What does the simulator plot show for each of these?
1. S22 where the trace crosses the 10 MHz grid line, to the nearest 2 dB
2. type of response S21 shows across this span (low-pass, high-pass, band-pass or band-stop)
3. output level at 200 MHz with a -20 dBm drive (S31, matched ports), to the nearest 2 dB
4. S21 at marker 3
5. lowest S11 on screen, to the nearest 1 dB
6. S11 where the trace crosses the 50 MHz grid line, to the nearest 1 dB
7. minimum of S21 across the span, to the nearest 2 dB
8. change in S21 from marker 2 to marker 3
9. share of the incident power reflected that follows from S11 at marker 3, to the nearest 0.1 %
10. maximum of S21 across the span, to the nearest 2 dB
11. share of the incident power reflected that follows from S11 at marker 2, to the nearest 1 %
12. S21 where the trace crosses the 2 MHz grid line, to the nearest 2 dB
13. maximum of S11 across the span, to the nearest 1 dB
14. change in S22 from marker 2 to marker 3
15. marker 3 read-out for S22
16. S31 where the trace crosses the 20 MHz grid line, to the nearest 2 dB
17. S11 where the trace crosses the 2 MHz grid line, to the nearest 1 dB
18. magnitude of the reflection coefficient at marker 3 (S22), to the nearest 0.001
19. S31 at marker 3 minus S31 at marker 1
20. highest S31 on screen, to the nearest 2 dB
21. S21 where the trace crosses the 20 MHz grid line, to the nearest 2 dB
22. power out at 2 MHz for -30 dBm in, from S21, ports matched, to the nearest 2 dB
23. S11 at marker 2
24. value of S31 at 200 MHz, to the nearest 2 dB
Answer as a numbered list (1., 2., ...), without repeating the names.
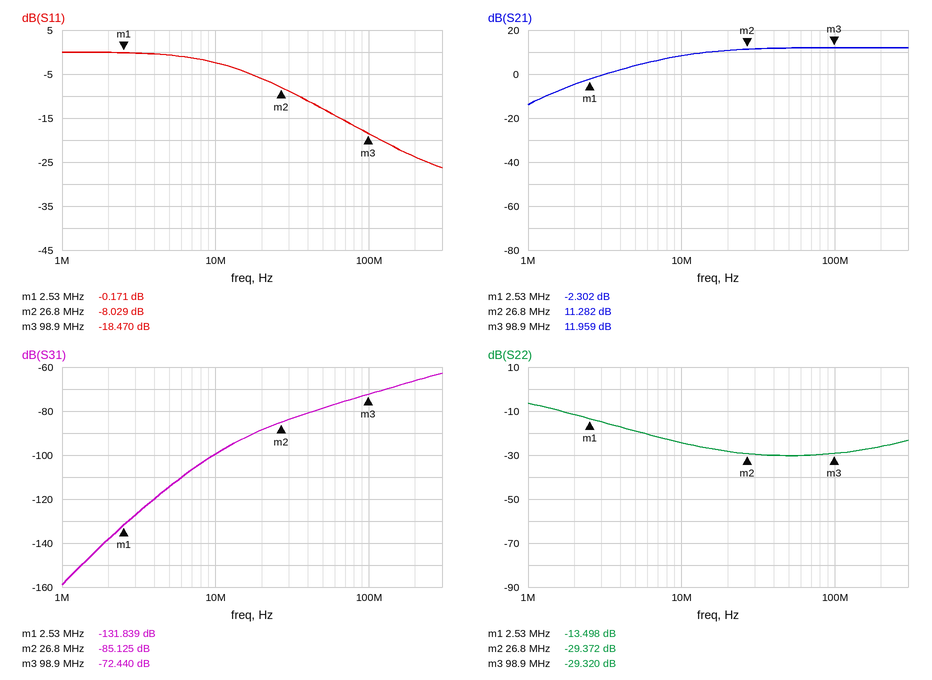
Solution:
1. -24 dB
2. high-pass
3. -86 dBm
4. 11.959 dB
5. -26 dB
6. -13 dB
7. -14 dB
8. 0.677 dB
9. 1.4 %
10. 12 dB
11. 16 %
12. -4 dB
13. 0 dB
14. 0.052 dB
15. -29.320 dB
16. -88 dB
17. 0 dB
18. 0.034
19. 59.399 dB
20. -62 dB
21. 10 dB
22. -34 dBm
23. -8.029 dB
24. -66 dB
